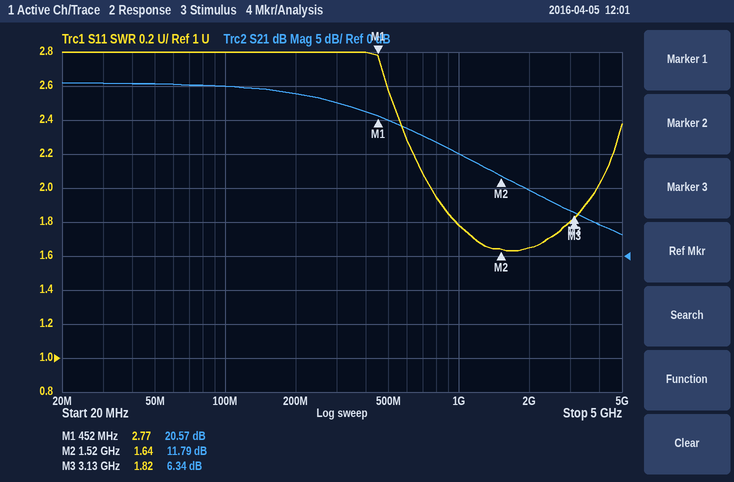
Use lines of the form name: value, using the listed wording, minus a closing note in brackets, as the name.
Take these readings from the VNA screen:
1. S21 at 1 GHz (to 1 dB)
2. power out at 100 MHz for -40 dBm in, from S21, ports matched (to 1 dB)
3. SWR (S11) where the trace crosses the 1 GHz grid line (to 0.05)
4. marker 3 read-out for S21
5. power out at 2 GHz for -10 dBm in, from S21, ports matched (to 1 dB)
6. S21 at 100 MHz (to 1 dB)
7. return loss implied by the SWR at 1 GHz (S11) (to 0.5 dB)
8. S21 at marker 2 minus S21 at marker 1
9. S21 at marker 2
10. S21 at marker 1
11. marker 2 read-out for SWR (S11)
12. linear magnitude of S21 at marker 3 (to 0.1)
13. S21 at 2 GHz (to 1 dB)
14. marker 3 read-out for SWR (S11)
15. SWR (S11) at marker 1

S21 at 1 GHz: 15 dB
power out at 100 MHz for -40 dBm in, from S21, ports matched: -15 dBm
SWR (S11) where the trace crosses the 1 GHz grid line: 1.80
marker 3 read-out for S21: 6.34 dB
power out at 2 GHz for -10 dBm in, from S21, ports matched: 0 dBm
S21 at 100 MHz: 25 dB
return loss implied by the SWR at 1 GHz (S11): 11.0 dB
S21 at marker 2 minus S21 at marker 1: -8.78 dB
S21 at marker 2: 11.79 dB
S21 at marker 1: 20.57 dB
marker 2 read-out for SWR: 1.64
linear magnitude of S21 at marker 3: 2.1
S21 at 2 GHz: 10 dB
marker 3 read-out for SWR: 1.82
SWR (S11) at marker 1: 2.77
